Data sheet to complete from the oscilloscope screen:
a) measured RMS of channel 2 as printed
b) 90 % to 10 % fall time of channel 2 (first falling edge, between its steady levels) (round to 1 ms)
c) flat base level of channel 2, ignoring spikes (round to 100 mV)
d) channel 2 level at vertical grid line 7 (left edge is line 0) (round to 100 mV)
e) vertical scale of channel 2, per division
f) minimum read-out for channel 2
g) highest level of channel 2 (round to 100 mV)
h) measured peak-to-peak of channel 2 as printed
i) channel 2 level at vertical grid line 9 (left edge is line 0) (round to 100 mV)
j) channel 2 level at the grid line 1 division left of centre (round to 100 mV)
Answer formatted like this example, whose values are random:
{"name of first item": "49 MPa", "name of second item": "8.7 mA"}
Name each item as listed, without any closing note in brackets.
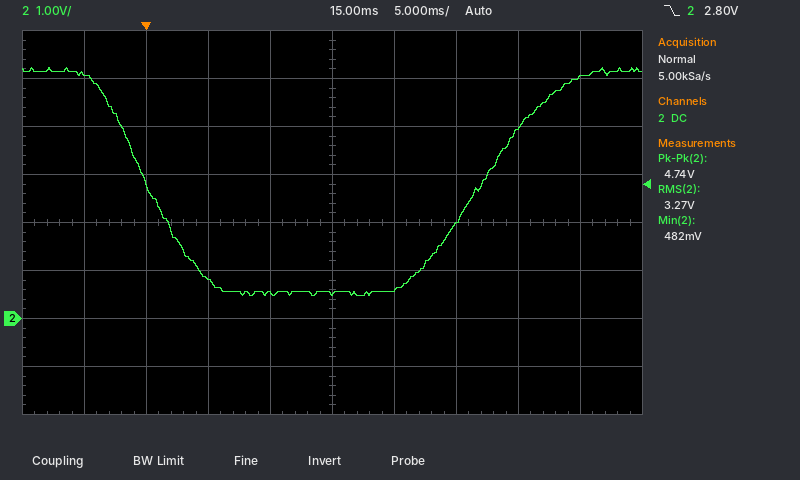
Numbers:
{"measured RMS of channel 2 as printed": "3.27 V", "90 % to 10 % fall time of channel 2 (first falling edge, between its steady levels)": "8 ms", "flat base level of channel 2, ignoring spikes": "600 mV", "channel 2 level at vertical grid line 7 (left edge is line 0)": "2.0 V", "vertical scale of channel 2, per division": "1 V", "minimum read-out for channel 2": "482 mV", "highest level of channel 2": "5.2 V", "measured peak-to-peak of channel 2 as printed": "4.74 V", "channel 2 level at vertical grid line 9 (left edge is line 0)": "5.0 V", "channel 2 level at the grid line 1 division left of centre": "500 mV"}
